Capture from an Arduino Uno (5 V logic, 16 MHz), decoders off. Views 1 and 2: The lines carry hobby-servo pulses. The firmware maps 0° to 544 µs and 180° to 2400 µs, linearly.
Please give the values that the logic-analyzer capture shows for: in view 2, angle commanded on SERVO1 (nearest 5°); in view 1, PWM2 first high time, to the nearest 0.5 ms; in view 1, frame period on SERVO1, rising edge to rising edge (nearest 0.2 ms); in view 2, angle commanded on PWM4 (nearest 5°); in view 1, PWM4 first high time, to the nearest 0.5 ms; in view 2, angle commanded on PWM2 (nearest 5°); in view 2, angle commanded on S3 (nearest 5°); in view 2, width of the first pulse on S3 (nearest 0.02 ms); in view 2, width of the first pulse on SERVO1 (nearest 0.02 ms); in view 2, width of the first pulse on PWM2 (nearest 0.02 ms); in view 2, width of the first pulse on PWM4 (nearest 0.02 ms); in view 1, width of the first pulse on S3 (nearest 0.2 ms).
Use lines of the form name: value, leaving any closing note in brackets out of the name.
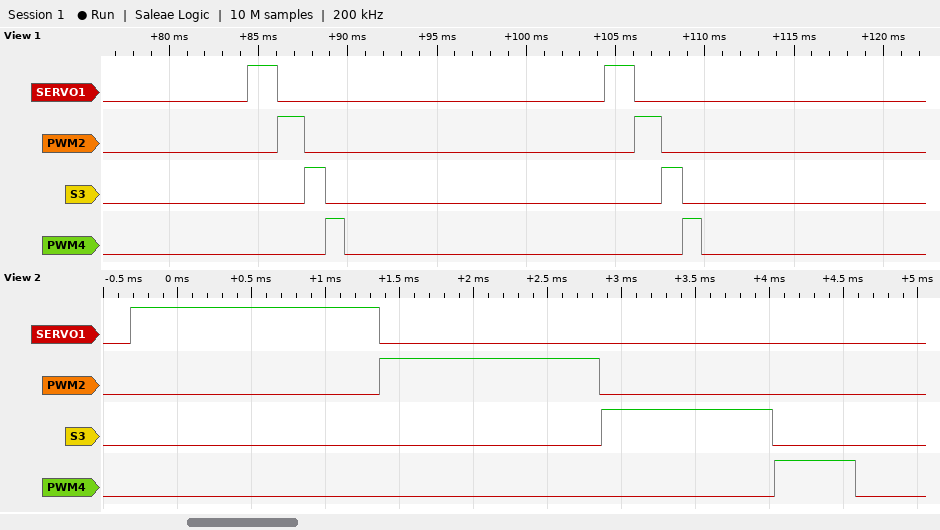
in view 2, angle commanded on SERVO1: 110°
in view 1, PWM2 first high time, to the nearest 0.5 ms: 1.5 ms
in view 1, frame period on SERVO1, rising edge to rising edge: 20.0 ms
in view 2, angle commanded on PWM4: 0°
in view 1, PWM4 first high time, to the nearest 0.5 ms: 1.0 ms
in view 2, angle commanded on PWM2: 90°
in view 2, angle commanded on S3: 60°
in view 2, width of the first pulse on S3: 1.16 ms
in view 2, width of the first pulse on SERVO1: 1.68 ms
in view 2, width of the first pulse on PWM2: 1.48 ms
in view 2, width of the first pulse on PWM4: 0.54 ms
in view 1, width of the first pulse on S3: 1.2 ms
